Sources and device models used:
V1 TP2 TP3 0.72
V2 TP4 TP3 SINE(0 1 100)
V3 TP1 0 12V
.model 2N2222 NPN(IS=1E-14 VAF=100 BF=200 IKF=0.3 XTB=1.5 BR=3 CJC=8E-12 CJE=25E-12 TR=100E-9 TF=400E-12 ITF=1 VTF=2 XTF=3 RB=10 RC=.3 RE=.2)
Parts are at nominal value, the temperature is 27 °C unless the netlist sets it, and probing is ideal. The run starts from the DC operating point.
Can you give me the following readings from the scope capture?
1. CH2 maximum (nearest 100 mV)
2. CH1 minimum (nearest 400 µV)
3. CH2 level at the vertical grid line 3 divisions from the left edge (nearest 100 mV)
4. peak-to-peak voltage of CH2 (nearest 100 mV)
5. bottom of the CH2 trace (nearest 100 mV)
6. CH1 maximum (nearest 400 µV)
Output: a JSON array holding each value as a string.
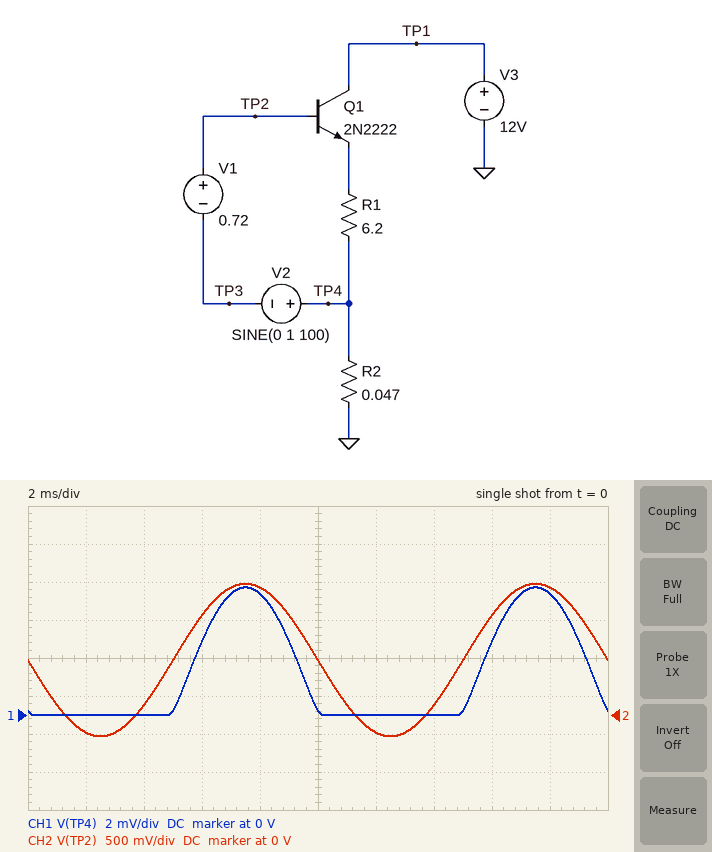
["1.7 V", "0 V", "1.3 V", "2.0 V", "-300 mV", "6.8 mV"]
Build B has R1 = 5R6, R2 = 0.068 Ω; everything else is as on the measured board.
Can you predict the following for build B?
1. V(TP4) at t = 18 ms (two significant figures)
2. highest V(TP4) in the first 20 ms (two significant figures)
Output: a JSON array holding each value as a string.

["10 mV", "11 mV"]
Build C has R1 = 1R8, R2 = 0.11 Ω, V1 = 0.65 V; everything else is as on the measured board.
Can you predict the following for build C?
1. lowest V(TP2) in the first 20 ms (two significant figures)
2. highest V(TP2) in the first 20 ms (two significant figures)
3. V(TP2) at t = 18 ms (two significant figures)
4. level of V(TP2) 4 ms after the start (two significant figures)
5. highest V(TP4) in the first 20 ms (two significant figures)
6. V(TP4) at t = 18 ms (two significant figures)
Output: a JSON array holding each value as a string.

["-350 mV", "1.7 V", "1.6 V", "62 mV", "43 mV", "40 mV"]
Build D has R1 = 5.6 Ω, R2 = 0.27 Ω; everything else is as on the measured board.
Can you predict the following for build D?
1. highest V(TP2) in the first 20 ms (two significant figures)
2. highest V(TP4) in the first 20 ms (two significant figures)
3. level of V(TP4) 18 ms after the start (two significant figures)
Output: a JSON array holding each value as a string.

["1.8 V", "42 mV", "40 mV"]
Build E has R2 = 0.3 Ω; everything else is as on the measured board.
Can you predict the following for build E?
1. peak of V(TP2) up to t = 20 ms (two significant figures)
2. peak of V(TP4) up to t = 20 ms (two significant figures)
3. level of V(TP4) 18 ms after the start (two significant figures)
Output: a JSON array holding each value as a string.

["1.8 V", "43 mV", "41 mV"]
